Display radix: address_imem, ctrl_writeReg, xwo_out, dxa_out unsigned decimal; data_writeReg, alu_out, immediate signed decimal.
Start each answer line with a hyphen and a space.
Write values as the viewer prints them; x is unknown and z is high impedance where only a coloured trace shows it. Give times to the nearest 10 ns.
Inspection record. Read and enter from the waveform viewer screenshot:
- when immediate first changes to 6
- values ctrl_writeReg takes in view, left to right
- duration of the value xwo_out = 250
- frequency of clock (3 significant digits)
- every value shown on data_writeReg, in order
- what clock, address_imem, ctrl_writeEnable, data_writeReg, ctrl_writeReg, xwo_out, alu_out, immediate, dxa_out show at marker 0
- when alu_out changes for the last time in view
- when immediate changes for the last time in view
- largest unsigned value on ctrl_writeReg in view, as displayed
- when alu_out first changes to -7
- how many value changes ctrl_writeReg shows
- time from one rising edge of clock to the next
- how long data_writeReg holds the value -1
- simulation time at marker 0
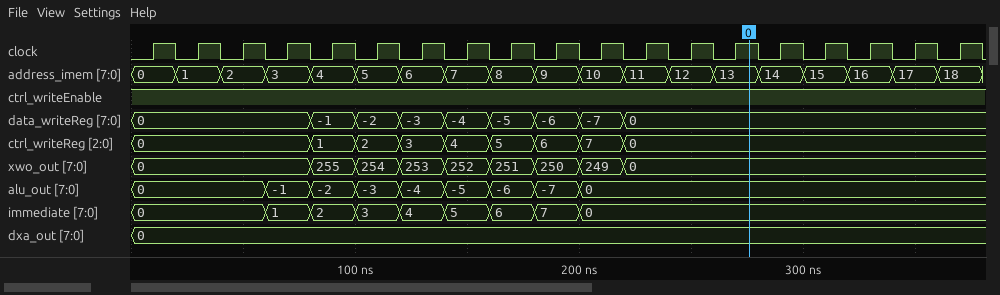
- 160 ns
- 0, 1, 2, 3, 4, 5, 6, 7, 0
- 20 ns
- 50.0 MHz
- 0, -1, -2, -3, -4, -5, -6, -7, 0
- clock=1, address_imem=13, ctrl_writeEnable=1, data_writeReg=0, ctrl_writeReg=0, xwo_out=0, alu_out=0, immediate=0, dxa_out=0
- 200 ns
- 200 ns
- 7
- 180 ns
- 8
- 20 ns
- 20 ns
- 280 ns
